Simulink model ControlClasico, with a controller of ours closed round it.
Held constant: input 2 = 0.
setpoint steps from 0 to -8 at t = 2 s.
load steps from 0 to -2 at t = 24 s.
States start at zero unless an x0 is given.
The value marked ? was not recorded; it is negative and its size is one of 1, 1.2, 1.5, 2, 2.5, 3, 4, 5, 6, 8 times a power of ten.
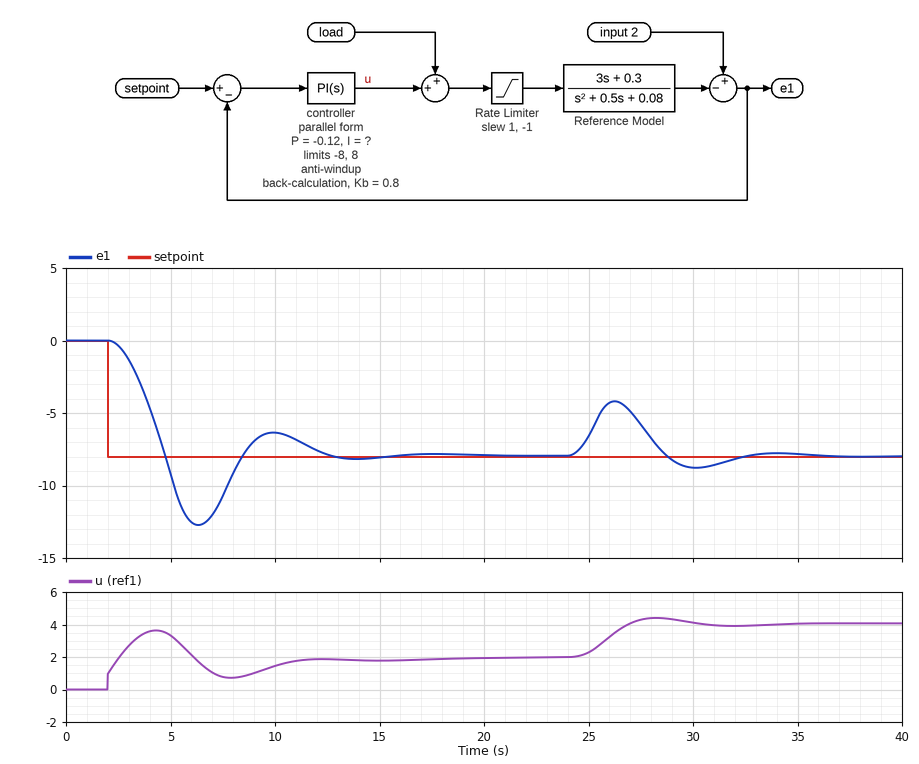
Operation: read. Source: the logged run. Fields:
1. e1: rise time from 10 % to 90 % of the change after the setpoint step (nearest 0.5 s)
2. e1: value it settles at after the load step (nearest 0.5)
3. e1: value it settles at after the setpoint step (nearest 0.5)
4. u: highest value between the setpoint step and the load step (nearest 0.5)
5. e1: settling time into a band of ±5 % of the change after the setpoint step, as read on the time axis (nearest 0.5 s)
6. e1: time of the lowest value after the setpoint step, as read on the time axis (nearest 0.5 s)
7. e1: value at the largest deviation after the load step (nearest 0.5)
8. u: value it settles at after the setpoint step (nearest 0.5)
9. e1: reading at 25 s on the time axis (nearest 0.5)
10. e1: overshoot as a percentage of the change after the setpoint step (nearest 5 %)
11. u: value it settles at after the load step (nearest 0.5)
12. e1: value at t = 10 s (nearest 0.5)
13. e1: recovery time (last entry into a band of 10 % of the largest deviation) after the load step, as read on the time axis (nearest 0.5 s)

2.0 s
-8.0
-8.0
3.5
12.0 s
6.5 s
-4.0
2.0
-6.5
60 %
4.0
-6.5
31.5 s
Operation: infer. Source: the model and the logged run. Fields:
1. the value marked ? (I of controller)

-0.25
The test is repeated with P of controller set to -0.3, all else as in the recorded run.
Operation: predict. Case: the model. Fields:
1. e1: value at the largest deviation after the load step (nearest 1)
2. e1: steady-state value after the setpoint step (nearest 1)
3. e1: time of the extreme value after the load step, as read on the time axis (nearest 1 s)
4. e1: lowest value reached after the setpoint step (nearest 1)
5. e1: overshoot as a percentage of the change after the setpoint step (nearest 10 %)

-5
-8
26 s
-12
50 %
